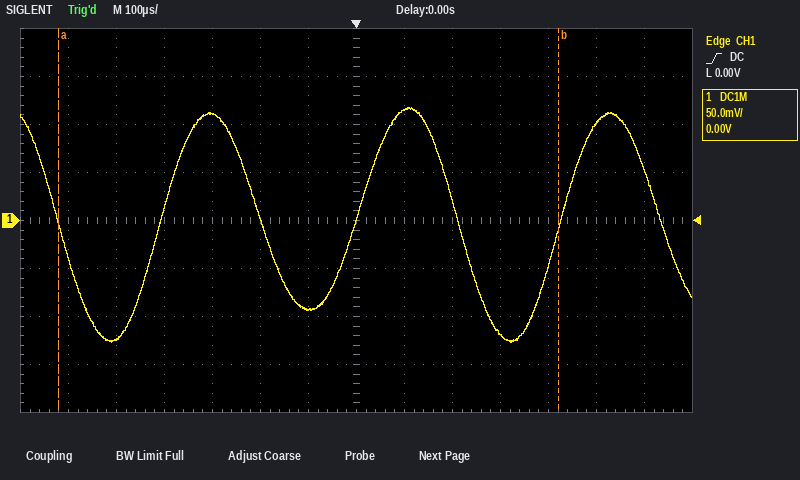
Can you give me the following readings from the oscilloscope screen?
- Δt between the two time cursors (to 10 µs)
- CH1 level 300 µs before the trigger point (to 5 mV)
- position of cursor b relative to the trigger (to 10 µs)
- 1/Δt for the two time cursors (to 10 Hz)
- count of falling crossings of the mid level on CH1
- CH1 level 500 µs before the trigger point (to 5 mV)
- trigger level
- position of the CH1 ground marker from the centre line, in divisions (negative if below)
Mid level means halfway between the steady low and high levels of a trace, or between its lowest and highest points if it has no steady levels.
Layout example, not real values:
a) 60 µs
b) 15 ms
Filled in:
a) 1.04 ms
b) 110 mV
c) +420 µs
d) 960 Hz
e) 4
f) -125 mV
g) 0.00 V
h) 0.0 div
